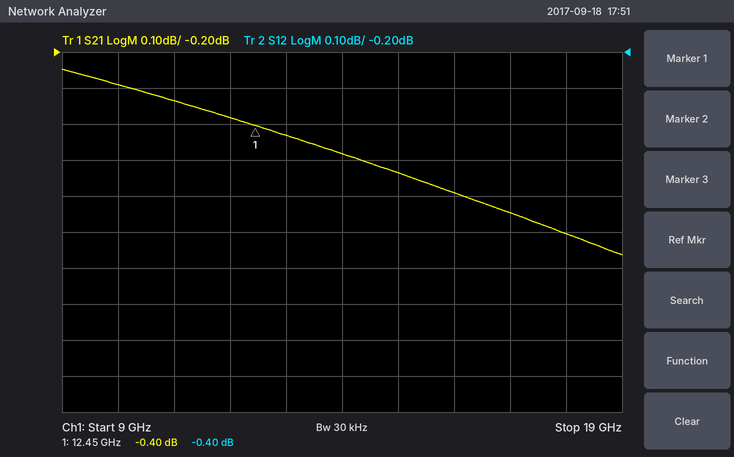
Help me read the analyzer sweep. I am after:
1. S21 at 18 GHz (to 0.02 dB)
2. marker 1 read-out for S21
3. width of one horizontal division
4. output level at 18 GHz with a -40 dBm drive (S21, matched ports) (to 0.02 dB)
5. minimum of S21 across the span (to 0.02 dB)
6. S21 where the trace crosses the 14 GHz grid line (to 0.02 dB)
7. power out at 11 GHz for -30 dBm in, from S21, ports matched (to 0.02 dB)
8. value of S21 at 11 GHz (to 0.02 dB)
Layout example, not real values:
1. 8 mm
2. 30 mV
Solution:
1. -0.70 dB
2. -0.40 dB
3. 1 GHz
4. -40.70 dBm
5. -0.76 dB
6. -0.48 dB
7. -30.34 dBm
8. -0.34 dB
